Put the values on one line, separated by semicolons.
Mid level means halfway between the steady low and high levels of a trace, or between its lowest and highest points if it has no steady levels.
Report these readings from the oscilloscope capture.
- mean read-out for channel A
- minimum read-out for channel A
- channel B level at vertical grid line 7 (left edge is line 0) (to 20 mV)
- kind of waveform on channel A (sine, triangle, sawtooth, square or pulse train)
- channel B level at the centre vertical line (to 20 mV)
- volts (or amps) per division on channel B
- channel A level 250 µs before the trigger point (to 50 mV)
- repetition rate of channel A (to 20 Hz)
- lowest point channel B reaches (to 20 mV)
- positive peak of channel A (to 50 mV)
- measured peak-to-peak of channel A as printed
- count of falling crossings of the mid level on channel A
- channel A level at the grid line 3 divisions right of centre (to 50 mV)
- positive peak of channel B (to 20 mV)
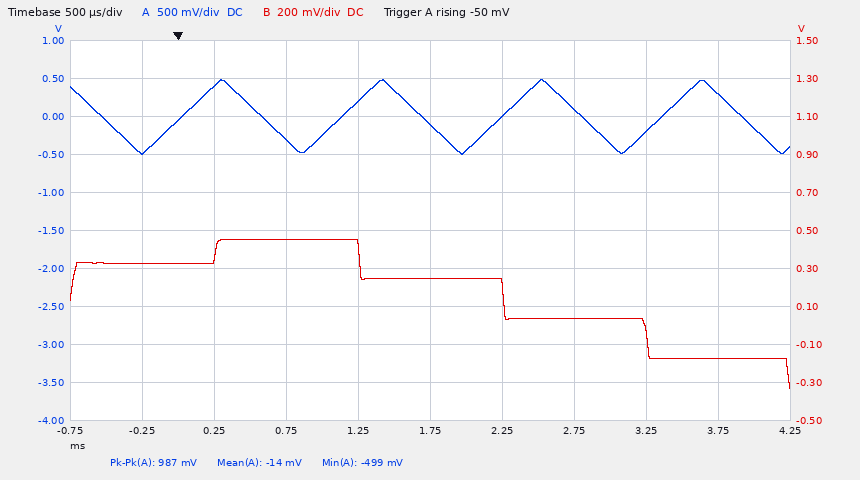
-14 mV; -499 mV; 40 mV; triangle; 240 mV; 200 mV; -500 mV; 900 Hz; -340 mV; 500 mV; 987 mV; 5; -200 mV; 460 mV
